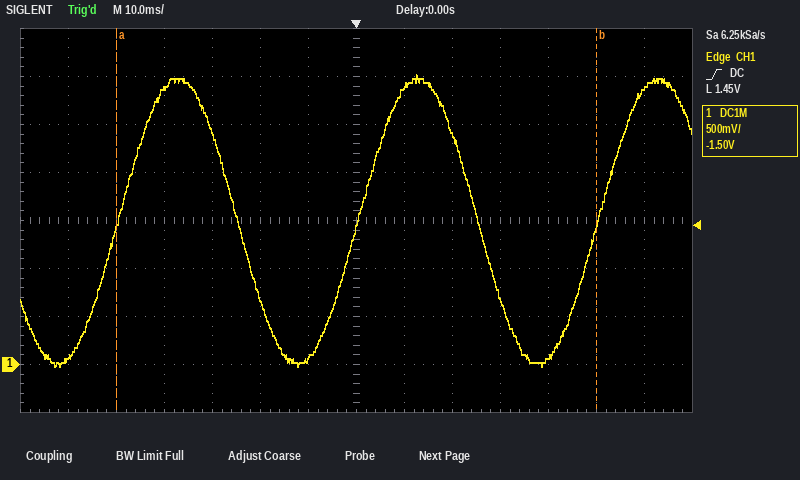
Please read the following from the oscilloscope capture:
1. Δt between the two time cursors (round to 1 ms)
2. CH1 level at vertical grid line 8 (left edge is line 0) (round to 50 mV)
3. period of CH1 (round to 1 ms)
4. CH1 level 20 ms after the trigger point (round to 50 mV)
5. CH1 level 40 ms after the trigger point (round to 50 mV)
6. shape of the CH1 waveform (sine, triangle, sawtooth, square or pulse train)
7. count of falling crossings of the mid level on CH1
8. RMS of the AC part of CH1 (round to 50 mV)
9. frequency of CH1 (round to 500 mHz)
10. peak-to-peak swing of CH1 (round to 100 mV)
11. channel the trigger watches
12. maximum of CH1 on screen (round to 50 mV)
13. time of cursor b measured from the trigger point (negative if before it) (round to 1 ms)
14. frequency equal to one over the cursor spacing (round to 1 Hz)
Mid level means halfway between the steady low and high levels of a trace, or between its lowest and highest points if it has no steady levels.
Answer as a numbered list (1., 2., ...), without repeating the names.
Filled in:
1. 100 ms
2. 2.90 V
3. 50 ms
4. 2.40 V
5. 100 mV
6. sine
7. 2
8. 1.05 V
9. 20.0 Hz
10. 3.00 V
11. CH1
12. 3.00 V
13. +50 ms
14. 10 Hz
